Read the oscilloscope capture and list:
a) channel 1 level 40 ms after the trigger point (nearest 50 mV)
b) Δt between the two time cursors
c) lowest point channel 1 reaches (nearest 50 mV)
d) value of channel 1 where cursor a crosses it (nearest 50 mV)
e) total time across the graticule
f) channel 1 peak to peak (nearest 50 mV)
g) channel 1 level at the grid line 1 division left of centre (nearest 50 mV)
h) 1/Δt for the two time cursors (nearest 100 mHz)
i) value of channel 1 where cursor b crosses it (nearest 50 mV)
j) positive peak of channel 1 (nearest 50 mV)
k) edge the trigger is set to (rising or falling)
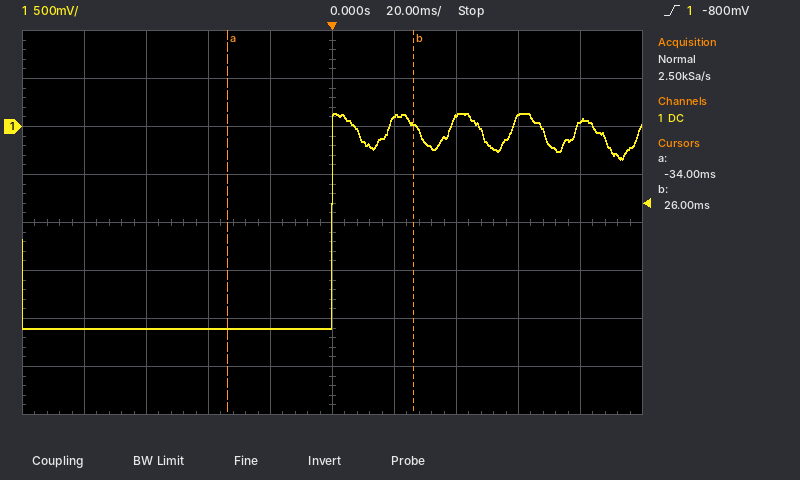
100 mV
60 ms
-2.10 V
-2.10 V
200 ms
2.25 V
-2.10 V
16.7 Hz
0 mV
150 mV
rising
